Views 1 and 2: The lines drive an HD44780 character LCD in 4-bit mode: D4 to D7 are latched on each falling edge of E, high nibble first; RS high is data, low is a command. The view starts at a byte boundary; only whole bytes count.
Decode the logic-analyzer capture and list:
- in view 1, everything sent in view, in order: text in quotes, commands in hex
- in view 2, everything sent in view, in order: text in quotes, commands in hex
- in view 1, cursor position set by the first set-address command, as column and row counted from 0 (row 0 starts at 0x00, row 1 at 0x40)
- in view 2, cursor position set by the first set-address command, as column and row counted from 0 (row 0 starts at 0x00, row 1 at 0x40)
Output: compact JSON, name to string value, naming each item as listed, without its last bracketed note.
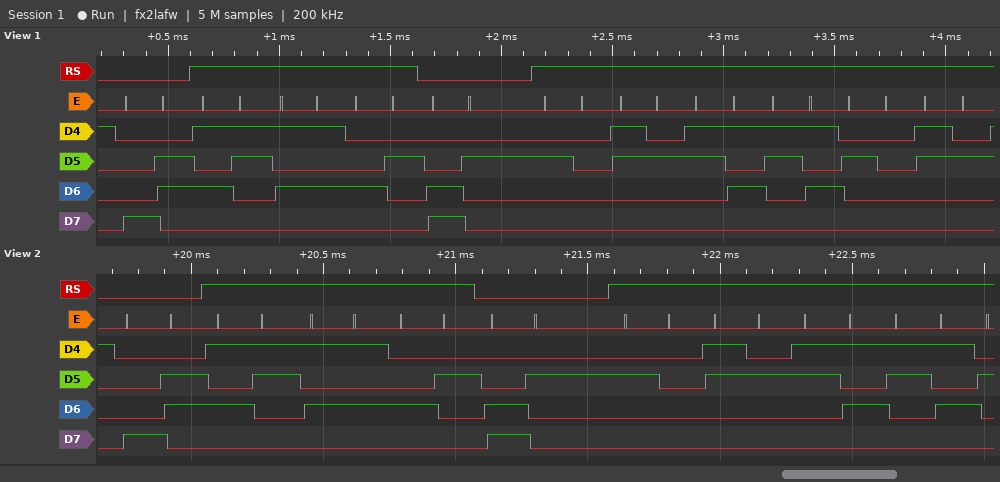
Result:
{"in view 1, everything sent in view, in order: text in quotes, commands in hex": "0x86 \"SUB\" 0xC2 \" 255 2\"", "in view 2, everything sent in view, in order: text in quotes, commands in hex": "0x86 \"SUB\" 0xC2 \" 255\"", "in view 1, cursor position set by the first set-address command, as column and row counted from 0": "column 6, row 0", "in view 2, cursor position set by the first set-address command, as column and row counted from 0": "column 6, row 0"}
